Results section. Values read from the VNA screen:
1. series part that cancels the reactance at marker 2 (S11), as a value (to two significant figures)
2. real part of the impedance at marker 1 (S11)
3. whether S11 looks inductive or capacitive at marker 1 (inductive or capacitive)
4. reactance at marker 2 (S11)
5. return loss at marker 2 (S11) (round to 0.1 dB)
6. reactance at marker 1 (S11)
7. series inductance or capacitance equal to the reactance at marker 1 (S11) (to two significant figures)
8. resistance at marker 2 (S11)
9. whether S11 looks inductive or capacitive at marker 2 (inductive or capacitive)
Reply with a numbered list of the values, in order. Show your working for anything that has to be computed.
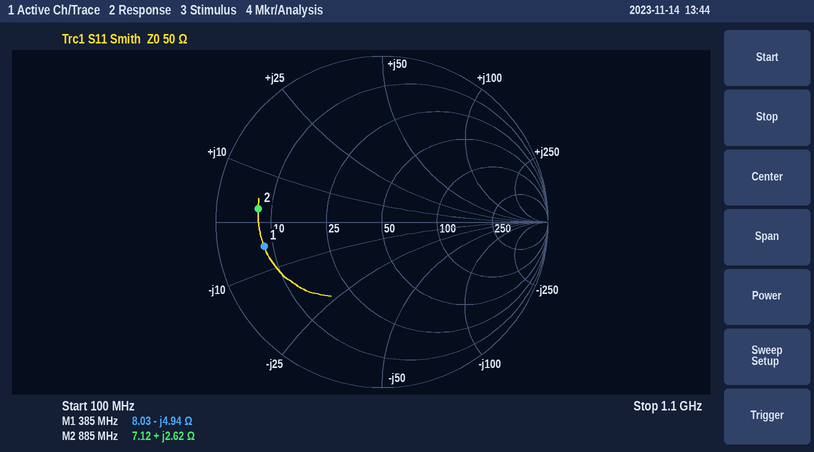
1. C = 1/(2π × 885 MHz × 2.62 Ω) ≈ 69 pF
2. 8.03 Ω
3. capacitive
4. +2.62 Ω
5. 2.5 dB
6. -4.94 Ω
7. C = 1/(2π × 385 MHz × 4.94 Ω) ≈ 84 pF
8. 7.12 Ω
9. inductive
